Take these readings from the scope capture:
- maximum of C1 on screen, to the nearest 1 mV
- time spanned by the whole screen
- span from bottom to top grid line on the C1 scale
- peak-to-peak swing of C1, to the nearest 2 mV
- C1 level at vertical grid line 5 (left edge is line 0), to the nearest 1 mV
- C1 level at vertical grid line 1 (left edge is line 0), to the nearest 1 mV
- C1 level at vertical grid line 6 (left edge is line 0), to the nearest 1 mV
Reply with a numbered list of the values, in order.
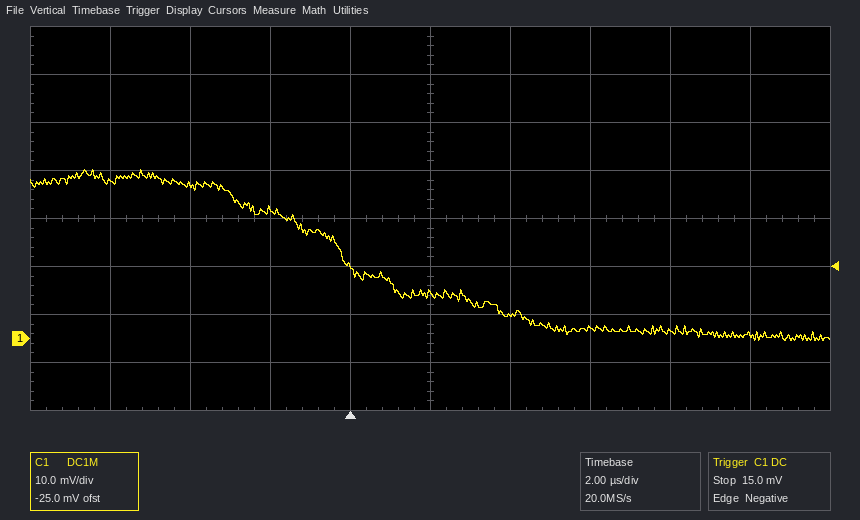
1. 35 mV
2. 20 µs
3. 80 mV
4. 36 mV
5. 9 mV
6. 33 mV
7. 5 mV
